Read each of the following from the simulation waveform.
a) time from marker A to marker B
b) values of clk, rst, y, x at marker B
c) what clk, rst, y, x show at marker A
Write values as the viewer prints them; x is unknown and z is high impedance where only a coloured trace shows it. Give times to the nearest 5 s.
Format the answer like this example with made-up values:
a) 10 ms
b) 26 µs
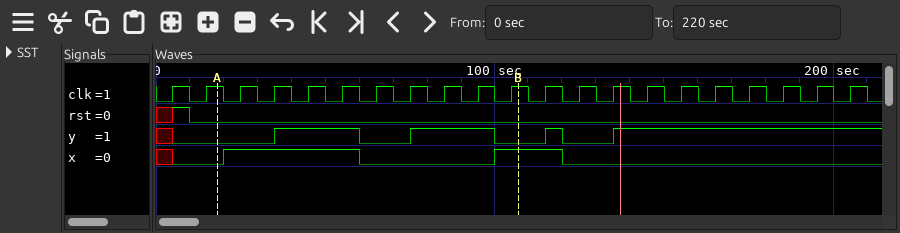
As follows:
a) 90 s
b) clk=1, rst=0, y=0, x=1
c) clk=1, rst=0, y=0, x=0
